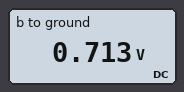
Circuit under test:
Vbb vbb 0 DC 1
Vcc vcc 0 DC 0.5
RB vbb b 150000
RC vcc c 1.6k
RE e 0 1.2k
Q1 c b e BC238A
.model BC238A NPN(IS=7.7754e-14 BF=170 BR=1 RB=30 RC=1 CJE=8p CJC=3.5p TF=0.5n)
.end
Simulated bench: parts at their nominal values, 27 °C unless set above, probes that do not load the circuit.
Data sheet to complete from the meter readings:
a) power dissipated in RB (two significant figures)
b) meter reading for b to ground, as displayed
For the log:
550 nW
0.713 V
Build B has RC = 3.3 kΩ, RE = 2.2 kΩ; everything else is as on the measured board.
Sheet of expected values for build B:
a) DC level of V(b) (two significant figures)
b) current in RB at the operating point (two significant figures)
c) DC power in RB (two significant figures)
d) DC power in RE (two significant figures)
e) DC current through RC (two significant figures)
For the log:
700 mV
2.0 µA
610 nW
12 µW
72 µA
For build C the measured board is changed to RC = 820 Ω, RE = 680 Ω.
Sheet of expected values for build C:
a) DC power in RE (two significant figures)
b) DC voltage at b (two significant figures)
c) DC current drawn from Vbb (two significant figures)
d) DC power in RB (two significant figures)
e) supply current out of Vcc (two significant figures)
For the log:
36 µW
720 mV
1.9 µA
520 nW
230 µA
